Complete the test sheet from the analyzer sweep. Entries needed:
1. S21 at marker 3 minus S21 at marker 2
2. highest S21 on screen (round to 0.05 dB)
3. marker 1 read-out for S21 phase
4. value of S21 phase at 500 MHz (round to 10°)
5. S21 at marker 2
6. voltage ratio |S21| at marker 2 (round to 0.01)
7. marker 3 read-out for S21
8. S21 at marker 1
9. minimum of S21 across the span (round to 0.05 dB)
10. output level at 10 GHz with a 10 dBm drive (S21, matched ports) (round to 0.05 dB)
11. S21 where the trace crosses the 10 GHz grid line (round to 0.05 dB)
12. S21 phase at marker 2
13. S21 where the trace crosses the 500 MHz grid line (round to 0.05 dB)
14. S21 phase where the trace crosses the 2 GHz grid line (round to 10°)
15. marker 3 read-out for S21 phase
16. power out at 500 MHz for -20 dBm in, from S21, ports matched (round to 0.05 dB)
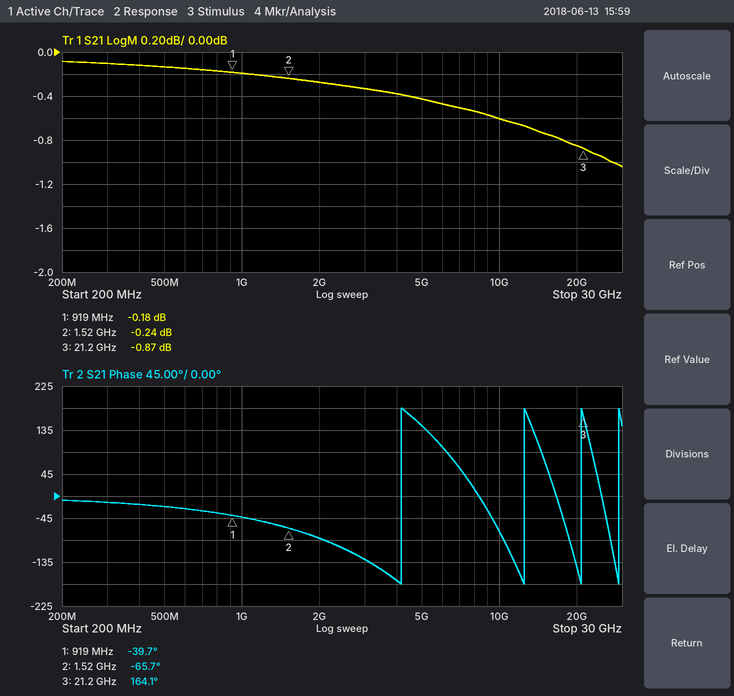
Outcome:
-0.63 dB
-0.10 dB
-39.7°
-20°
-0.24 dB
0.97
-0.87 dB
-0.18 dB
-1.05 dB
9.40 dBm
-0.60 dB
-65.7°
-0.15 dB
-90°
164.1°
-20.15 dBm
